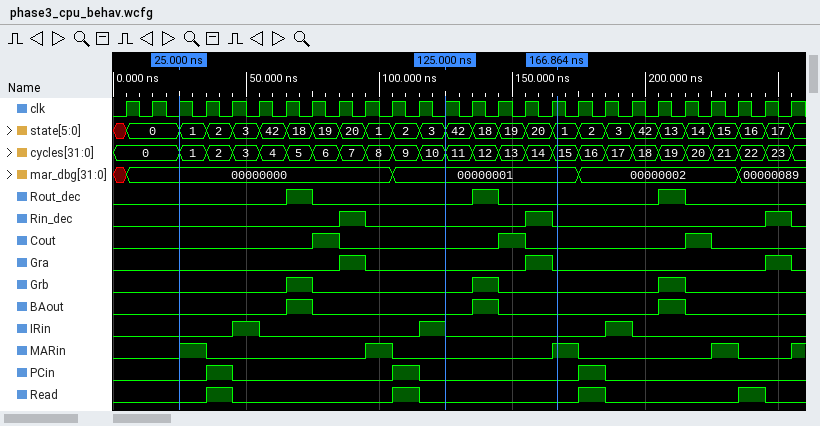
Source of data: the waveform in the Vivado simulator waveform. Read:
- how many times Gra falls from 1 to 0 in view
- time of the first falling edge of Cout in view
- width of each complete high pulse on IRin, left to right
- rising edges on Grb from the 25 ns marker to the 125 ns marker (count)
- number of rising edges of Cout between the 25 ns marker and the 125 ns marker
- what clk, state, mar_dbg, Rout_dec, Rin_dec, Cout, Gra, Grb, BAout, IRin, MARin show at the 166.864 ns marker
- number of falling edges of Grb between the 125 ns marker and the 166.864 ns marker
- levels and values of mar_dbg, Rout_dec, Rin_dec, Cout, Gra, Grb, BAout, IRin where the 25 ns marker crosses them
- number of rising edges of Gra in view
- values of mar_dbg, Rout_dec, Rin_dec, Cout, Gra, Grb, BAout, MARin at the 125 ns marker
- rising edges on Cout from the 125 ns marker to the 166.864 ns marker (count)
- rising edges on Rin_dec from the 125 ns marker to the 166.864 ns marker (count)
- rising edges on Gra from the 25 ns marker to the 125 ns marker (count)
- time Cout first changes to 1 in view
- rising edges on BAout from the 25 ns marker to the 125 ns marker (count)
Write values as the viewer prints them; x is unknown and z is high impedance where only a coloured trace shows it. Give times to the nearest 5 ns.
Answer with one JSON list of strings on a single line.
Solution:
["3", "85 ns", "10 ns, 10 ns, 10 ns", "1", "1", "clk=1, state=1, mar_dbg=00000001, Rout_dec=0, Rin_dec=0, Cout=0, Gra=0, Grb=0, BAout=0, IRin=0, MARin=1", "1", "mar_dbg=00000000, Rout_dec=0, Rin_dec=0, Cout=0, Gra=0, Grb=0, BAout=0, IRin=0", "3", "mar_dbg=00000001, Rout_dec=0, Rin_dec=0, Cout=0, Gra=0, Grb=0, BAout=0, MARin=0", "1", "1", "1", "75 ns", "1"]
